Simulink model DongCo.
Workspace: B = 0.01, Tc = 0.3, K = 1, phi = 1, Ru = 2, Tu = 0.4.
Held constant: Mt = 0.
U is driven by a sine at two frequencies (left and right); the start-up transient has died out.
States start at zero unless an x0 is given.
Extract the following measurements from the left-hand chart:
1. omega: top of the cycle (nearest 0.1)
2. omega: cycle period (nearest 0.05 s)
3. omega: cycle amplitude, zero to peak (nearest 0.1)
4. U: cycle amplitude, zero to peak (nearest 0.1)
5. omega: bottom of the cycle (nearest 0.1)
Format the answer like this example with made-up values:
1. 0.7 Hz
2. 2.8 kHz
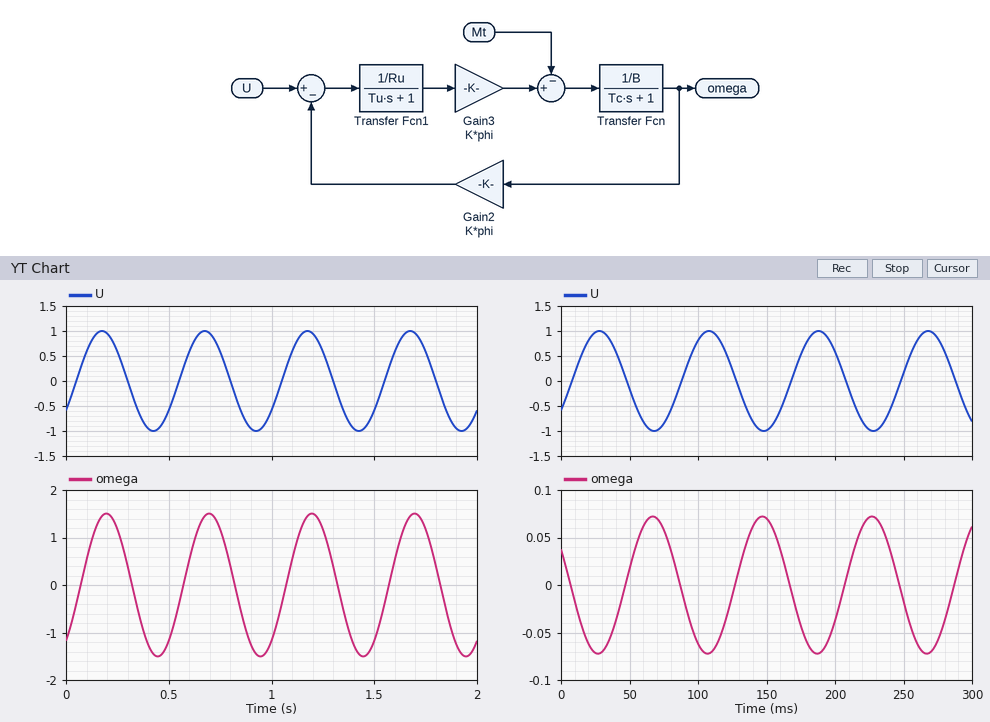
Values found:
1. 1.5
2. 0.50 s
3. 1.5
4. 1.0
5. -1.5
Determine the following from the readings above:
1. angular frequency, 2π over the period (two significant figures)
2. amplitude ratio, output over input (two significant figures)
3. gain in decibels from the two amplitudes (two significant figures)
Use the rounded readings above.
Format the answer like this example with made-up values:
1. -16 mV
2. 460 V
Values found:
1. 13 rad/s
2. 1.5
3. 3.5 dB
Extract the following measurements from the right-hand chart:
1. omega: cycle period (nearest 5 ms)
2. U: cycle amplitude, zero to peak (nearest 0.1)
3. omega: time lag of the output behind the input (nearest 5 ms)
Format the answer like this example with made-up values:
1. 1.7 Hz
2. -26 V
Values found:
1. 80 ms
2. 1.0
3. 40 ms
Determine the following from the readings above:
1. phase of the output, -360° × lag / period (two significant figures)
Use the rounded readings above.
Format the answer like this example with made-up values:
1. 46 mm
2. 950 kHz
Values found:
1. -180°
